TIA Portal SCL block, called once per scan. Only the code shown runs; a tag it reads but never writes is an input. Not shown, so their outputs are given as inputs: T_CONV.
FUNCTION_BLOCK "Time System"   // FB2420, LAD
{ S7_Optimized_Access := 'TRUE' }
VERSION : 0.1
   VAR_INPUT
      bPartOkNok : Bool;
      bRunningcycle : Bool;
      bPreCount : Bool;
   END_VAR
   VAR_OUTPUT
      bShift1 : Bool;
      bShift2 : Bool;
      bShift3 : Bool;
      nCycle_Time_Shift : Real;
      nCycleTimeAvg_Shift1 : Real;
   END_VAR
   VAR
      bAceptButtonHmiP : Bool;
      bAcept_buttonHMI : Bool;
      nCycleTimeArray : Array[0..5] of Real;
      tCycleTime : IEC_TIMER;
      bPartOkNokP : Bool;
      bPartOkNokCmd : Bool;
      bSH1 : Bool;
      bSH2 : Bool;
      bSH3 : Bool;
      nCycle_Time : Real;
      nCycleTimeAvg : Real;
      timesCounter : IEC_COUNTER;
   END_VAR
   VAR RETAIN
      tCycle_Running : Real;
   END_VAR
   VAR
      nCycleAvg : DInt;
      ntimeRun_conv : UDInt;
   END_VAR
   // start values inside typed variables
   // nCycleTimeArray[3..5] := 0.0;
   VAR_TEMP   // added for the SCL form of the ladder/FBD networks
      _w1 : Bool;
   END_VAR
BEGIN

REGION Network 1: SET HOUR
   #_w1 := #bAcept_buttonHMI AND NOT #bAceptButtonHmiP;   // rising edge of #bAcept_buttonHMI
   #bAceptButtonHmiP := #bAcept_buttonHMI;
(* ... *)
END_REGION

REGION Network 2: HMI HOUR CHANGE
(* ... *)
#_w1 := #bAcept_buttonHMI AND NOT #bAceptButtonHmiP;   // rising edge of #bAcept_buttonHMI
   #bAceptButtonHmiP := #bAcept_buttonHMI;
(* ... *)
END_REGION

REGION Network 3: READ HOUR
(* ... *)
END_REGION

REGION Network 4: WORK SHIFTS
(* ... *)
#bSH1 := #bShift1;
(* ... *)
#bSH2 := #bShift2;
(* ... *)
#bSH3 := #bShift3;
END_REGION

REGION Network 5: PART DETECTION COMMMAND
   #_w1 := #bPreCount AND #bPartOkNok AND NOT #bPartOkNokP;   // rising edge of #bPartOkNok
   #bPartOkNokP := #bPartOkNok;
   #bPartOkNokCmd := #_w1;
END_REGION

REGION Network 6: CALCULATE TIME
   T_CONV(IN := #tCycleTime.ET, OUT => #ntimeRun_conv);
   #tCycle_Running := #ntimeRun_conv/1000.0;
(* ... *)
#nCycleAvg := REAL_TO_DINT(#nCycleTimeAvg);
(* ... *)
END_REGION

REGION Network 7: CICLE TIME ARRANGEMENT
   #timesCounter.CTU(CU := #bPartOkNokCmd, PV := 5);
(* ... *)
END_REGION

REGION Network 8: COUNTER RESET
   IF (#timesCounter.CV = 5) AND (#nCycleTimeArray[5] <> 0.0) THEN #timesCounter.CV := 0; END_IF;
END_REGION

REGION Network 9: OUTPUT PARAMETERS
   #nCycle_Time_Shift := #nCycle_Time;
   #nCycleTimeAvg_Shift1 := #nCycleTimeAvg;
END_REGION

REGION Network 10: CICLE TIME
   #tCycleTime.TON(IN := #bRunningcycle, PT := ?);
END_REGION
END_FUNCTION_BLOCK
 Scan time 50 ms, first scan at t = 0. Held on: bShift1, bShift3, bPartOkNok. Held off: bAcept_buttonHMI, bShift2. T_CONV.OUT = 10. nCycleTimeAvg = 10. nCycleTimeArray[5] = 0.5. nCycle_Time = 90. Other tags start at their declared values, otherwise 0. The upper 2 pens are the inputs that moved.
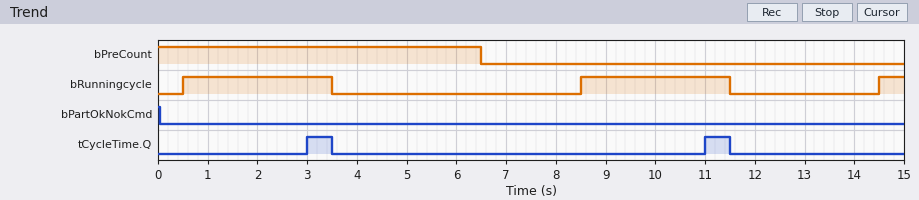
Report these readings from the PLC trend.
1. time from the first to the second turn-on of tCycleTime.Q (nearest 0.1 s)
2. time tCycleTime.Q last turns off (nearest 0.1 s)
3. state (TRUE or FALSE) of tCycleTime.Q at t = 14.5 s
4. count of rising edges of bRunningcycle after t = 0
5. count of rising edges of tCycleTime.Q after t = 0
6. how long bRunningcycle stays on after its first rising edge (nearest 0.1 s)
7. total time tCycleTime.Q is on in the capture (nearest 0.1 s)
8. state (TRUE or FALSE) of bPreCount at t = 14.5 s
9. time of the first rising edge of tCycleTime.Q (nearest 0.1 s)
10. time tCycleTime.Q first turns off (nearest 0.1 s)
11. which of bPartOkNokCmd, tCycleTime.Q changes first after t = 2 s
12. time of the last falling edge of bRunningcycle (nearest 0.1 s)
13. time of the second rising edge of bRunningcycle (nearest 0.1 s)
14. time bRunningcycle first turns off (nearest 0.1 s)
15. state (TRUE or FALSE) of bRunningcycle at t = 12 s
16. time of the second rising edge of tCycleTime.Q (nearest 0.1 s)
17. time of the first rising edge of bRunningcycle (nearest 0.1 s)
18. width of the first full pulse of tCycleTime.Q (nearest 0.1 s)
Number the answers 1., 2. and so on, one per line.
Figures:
1. 8.0 s
2. 11.5 s
3. FALSE
4. 3
5. 2
6. 3.0 s
7. 1.0 s
8. FALSE
9. 3.0 s
10. 3.5 s
11. tCycleTime.Q
12. 11.5 s
13. 8.5 s
14. 3.5 s
15. FALSE
16. 11.0 s
17. 0.5 s
18. 0.5 s
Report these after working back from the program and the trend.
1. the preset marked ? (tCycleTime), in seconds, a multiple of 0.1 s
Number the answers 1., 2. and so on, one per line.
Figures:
1. 2.5 s
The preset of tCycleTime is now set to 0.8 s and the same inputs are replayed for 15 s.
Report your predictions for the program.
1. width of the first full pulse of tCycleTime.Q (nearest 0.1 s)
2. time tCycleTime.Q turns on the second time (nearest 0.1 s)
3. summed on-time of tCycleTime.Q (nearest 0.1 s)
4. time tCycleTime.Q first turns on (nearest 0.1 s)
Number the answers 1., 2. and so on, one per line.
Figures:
1. 2.2 s
2. 9.3 s
3. 4.4 s
4. 1.3 s
